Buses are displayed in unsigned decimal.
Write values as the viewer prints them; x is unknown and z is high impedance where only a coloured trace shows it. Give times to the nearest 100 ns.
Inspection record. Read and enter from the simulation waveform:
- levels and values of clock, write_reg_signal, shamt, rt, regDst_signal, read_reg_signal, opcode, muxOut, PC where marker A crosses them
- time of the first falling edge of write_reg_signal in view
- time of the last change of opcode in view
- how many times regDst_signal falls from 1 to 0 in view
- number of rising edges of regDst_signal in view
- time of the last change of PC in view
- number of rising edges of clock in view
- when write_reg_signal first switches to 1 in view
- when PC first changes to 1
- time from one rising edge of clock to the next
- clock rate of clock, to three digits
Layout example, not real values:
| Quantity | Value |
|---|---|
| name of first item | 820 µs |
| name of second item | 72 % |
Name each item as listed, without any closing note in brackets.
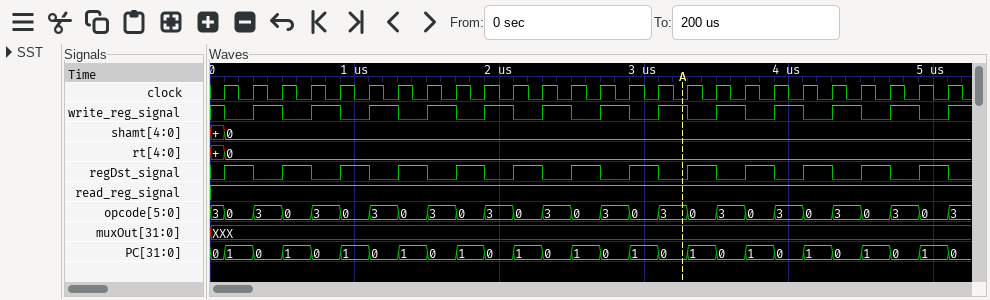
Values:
| Quantity | Value |
|---|---|
| levels and values of clock, write_reg_signal, shamt, rt, regDst_signal, read_reg_signal, opcode, muxOut, PC where marker A crosses them | clock=0, write_reg_signal=1, shamt=0, rt=0, regDst_signal=0, read_reg_signal=1, opcode=3, muxOut=XXX, PC=0 |
| time of the first falling edge of write_reg_signal in view | 100 ns |
| time of the last change of opcode in view | 5100 ns |
| how many times regDst_signal falls from 1 to 0 in view | 13 |
| number of rising edges of regDst_signal in view | 13 |
| time of the last change of PC in view | 5100 ns |
| number of rising edges of clock in view | 26 |
| when write_reg_signal first switches to 1 in view | 300 ns |
| when PC first changes to 1 | 100 ns |
| time from one rising edge of clock to the next | 200 ns |
| clock rate of clock, to three digits | 5.00 MHz |
